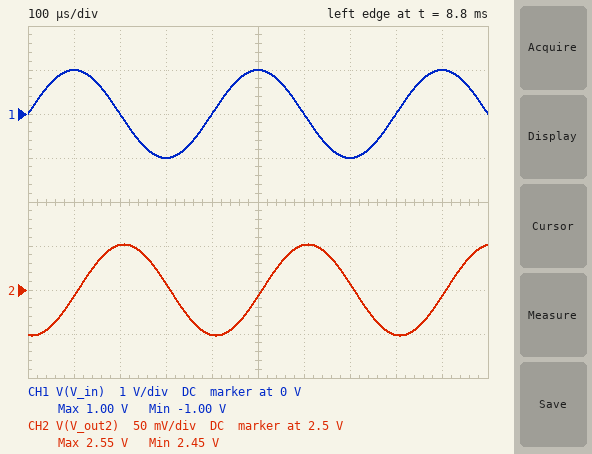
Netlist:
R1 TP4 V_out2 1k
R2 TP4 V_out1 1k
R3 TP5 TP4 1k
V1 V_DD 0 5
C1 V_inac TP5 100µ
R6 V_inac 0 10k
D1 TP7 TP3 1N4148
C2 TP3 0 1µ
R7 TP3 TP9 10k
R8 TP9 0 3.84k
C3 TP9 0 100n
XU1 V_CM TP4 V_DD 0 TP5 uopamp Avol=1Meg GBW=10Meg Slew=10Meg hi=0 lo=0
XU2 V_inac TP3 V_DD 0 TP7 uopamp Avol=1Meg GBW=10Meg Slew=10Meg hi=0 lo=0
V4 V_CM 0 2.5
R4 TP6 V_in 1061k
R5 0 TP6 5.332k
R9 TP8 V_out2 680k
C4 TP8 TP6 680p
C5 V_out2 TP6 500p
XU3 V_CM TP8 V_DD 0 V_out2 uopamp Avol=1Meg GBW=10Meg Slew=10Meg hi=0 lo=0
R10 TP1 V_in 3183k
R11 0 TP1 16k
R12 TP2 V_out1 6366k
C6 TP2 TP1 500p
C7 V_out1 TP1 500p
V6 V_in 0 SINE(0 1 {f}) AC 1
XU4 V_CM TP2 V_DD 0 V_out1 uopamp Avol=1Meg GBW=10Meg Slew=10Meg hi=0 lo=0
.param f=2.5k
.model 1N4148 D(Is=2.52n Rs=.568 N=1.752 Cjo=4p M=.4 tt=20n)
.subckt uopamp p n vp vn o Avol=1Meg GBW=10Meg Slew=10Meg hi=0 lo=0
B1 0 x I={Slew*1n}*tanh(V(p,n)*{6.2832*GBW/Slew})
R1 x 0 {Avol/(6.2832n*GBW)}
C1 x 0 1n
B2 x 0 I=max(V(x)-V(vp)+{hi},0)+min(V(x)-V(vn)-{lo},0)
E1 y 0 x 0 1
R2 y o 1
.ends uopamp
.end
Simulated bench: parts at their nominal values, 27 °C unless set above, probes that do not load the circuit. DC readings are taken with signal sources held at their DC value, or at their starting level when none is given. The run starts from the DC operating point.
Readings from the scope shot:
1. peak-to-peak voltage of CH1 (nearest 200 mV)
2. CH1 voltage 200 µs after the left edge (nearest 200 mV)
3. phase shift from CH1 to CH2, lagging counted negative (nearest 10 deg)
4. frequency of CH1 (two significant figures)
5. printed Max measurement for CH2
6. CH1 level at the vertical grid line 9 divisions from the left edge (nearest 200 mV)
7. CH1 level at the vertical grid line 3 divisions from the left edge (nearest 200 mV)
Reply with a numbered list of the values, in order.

1. 2.0 V
2. 0 V
3. -100 deg
4. 2.5 kHz
5. 2.55 V
6. 1.0 V
7. -1.0 V
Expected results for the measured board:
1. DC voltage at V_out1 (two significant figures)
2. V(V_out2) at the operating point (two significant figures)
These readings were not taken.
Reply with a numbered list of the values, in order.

1. 2.5 V
2. 2.5 V
